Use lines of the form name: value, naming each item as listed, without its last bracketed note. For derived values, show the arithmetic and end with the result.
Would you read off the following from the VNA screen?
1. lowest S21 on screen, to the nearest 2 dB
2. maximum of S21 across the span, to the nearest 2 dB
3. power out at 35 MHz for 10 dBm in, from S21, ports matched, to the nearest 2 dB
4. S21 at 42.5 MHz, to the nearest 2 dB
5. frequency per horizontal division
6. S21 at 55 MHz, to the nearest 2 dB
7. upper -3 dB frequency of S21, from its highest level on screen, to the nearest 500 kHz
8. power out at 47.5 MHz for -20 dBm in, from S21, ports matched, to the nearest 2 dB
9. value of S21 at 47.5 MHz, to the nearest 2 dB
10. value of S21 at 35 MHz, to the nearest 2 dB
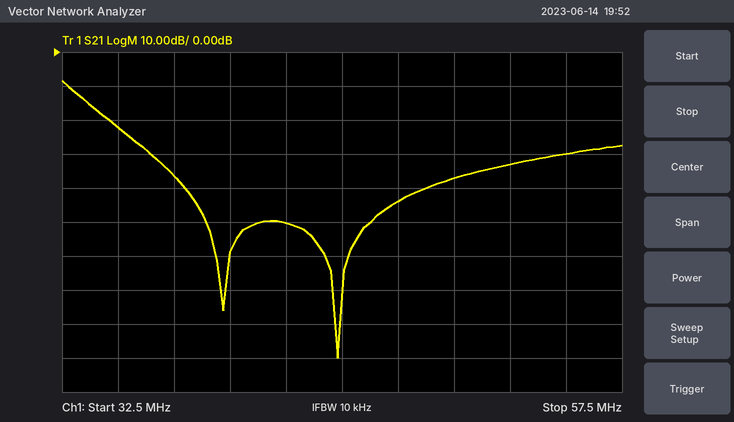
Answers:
lowest S21 on screen, to the nearest 2 dB: -90 dB
maximum of S21 across the span, to the nearest 2 dB: -8 dB
power out at 35 MHz for 10 dBm in, from S21, ports matched, to the nearest 2 dB: 10 dBm + (-22 dB) = -12 dBm
S21 at 42.5 MHz, to the nearest 2 dB: -50 dB
frequency per horizontal division: 2.5 MHz
S21 at 55 MHz, to the nearest 2 dB: -30 dB
upper -3 dB frequency of S21, from its highest level on screen, to the nearest 500 kHz: 33.0 MHz
power out at 47.5 MHz for -20 dBm in, from S21, ports matched, to the nearest 2 dB: -20 dBm + (-44 dB) = -64 dBm
value of S21 at 47.5 MHz, to the nearest 2 dB: -44 dB
value of S21 at 35 MHz, to the nearest 2 dB: -22 dB
